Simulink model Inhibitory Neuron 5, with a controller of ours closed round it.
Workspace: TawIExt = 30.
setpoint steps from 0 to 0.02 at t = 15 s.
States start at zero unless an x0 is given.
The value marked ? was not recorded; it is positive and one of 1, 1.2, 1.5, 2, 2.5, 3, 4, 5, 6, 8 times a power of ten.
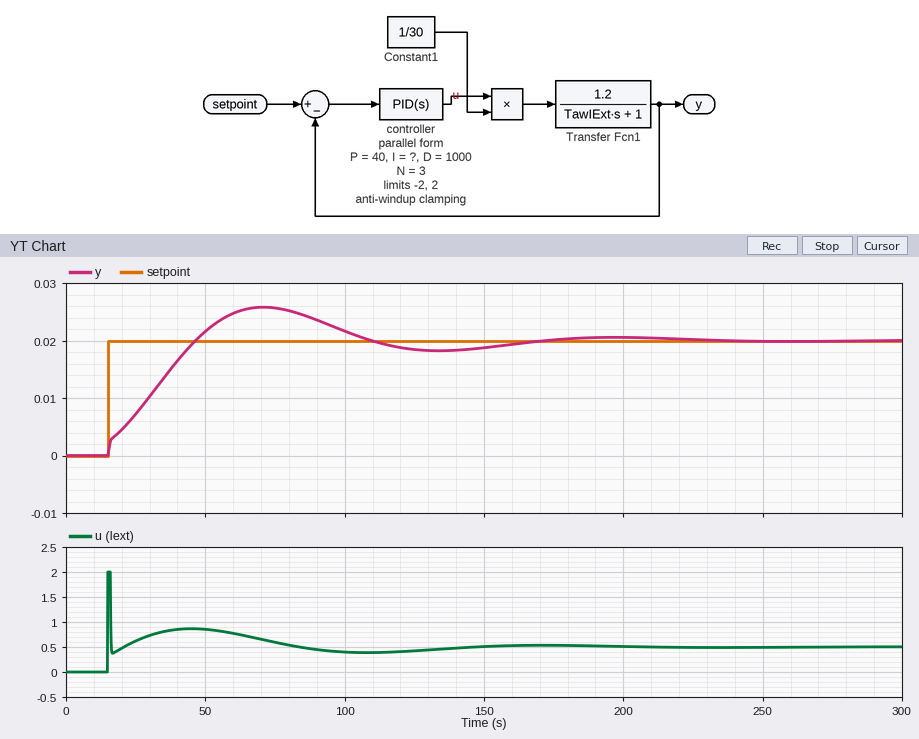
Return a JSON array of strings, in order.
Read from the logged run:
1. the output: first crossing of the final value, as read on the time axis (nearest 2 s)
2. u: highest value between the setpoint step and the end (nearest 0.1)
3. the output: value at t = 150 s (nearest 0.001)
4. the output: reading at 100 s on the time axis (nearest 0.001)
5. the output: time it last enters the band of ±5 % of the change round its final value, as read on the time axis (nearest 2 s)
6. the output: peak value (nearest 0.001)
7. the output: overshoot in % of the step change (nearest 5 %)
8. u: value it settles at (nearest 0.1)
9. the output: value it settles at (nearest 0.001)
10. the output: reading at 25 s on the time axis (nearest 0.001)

["46 s", "2.0", "0.019", "0.022", "154 s", "0.026", "30 %", "0.5", "0.020", "0.007"]
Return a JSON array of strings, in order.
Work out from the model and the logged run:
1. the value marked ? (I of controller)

["5"]
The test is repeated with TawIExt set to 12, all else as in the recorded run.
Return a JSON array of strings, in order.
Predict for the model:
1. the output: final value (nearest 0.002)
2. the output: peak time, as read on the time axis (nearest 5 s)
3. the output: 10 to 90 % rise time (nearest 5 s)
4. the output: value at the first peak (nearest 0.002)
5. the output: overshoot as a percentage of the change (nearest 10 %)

["0.020", "65 s", "25 s", "0.024", "20 %"]
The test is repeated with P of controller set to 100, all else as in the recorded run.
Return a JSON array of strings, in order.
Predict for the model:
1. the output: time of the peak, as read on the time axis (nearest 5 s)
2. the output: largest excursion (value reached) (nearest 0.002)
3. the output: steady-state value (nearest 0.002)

["65 s", "0.022", "0.020"]
